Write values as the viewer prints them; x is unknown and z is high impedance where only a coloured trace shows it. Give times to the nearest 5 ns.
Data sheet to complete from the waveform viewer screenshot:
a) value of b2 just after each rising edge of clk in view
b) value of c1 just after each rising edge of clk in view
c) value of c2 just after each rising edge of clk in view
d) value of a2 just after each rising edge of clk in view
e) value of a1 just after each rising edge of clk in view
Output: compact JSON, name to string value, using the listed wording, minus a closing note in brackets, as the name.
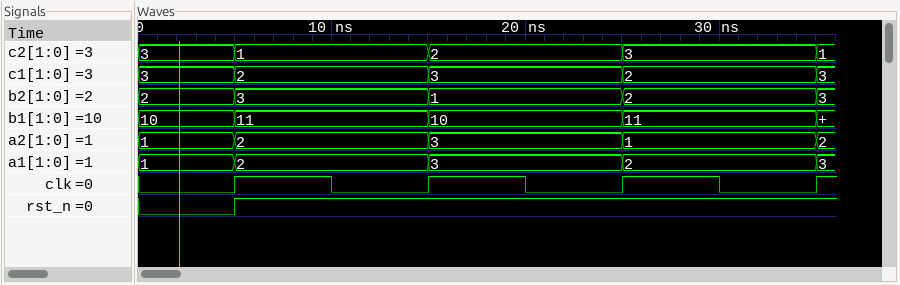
{"value of b2 just after each rising edge of clk in view": "3, 1, 2, 3", "value of c1 just after each rising edge of clk in view": "2, 3, 2, 3", "value of c2 just after each rising edge of clk in view": "1, 2, 3, 1", "value of a2 just after each rising edge of clk in view": "2, 3, 1, 2", "value of a1 just after each rising edge of clk in view": "2, 3, 2, 3"}
